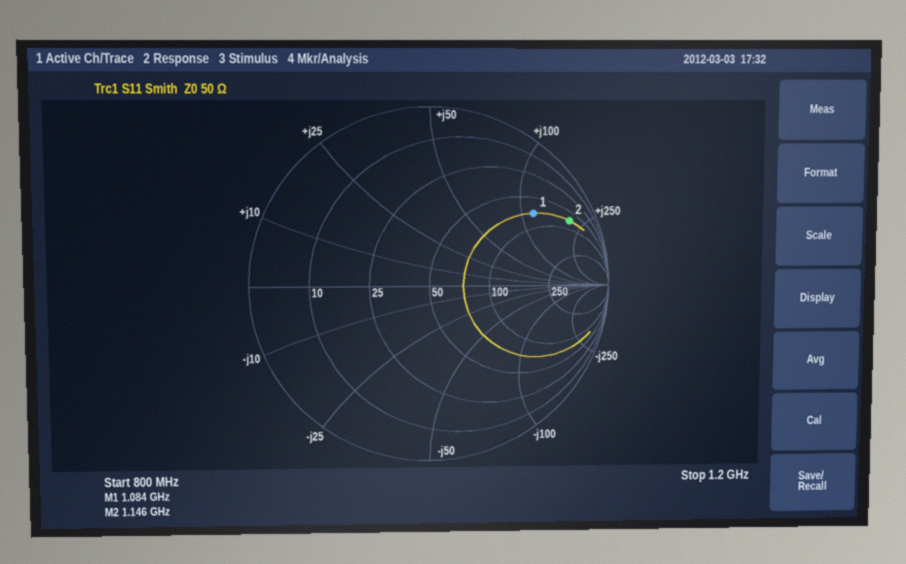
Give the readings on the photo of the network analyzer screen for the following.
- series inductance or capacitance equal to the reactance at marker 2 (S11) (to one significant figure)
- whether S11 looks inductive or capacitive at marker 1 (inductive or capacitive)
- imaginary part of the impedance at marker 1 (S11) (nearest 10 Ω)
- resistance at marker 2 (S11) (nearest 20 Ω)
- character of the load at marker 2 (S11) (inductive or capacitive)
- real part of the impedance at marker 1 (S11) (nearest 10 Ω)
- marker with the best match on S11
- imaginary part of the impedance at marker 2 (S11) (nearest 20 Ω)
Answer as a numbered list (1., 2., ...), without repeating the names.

1. 30 nH
2. inductive
3. +120 Ω
4. 80 Ω
5. inductive
6. 70 Ω
7. marker 1
8. +200 Ω
